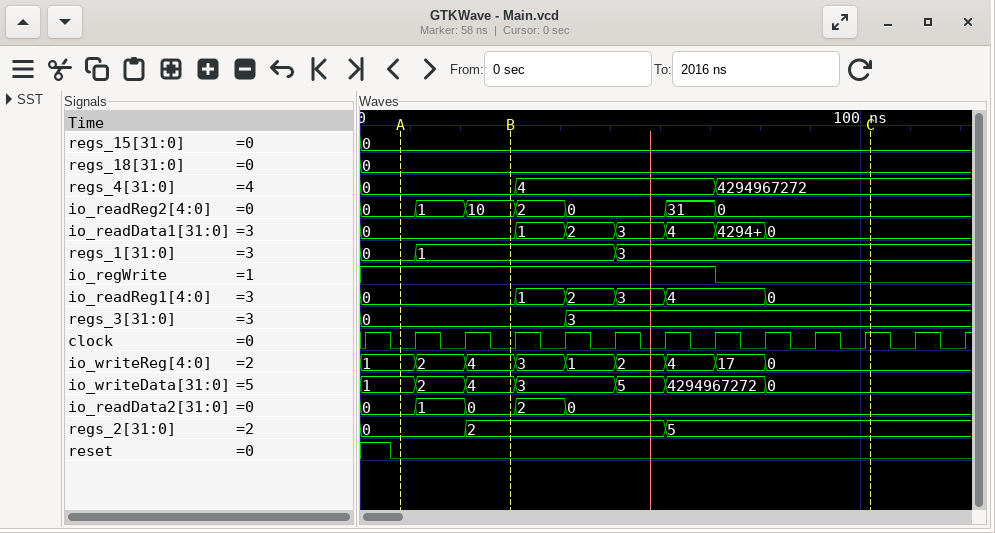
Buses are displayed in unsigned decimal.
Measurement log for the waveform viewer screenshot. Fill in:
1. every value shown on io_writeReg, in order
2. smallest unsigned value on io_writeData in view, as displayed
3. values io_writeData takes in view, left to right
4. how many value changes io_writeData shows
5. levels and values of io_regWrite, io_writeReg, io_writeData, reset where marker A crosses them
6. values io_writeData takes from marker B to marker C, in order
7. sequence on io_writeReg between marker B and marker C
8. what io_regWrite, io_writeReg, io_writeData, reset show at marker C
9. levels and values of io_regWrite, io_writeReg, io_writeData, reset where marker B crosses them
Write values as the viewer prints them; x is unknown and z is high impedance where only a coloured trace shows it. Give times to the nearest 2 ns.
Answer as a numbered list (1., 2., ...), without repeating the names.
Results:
1. 1, 2, 4, 3, 1, 2, 4, 17, 0
2. 0
3. 1, 2, 4, 3, 5, 4294967272, 0
4. 6
5. io_regWrite=1, io_writeReg=1, io_writeData=1, reset=0
6. 4, 3, 5, 4294967272, 0
7. 4, 3, 1, 2, 4, 17, 0
8. io_regWrite=0, io_writeReg=0, io_writeData=0, reset=0
9. io_regWrite=1, io_writeReg=4, io_writeData=4, reset=0
